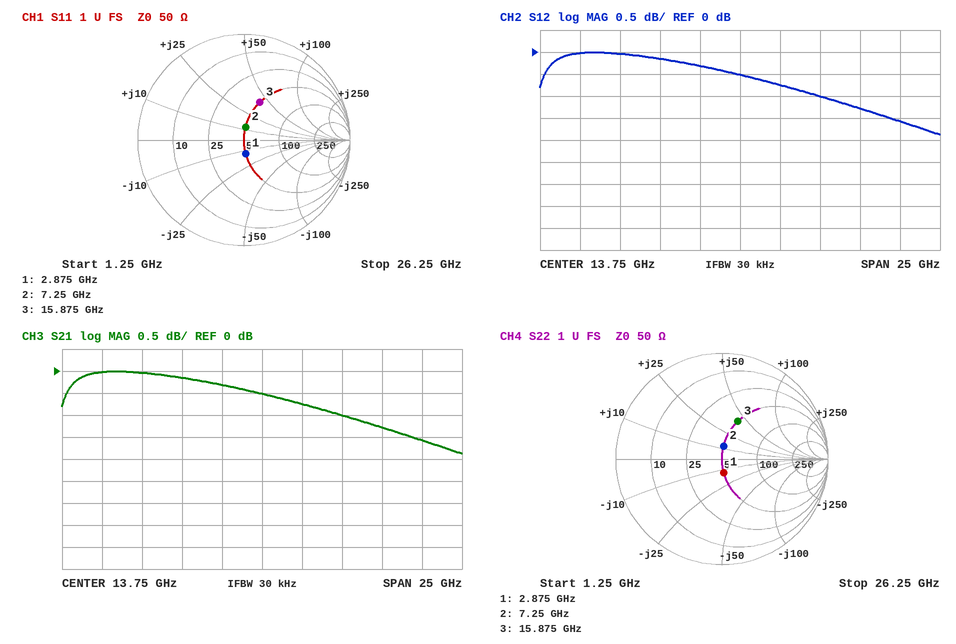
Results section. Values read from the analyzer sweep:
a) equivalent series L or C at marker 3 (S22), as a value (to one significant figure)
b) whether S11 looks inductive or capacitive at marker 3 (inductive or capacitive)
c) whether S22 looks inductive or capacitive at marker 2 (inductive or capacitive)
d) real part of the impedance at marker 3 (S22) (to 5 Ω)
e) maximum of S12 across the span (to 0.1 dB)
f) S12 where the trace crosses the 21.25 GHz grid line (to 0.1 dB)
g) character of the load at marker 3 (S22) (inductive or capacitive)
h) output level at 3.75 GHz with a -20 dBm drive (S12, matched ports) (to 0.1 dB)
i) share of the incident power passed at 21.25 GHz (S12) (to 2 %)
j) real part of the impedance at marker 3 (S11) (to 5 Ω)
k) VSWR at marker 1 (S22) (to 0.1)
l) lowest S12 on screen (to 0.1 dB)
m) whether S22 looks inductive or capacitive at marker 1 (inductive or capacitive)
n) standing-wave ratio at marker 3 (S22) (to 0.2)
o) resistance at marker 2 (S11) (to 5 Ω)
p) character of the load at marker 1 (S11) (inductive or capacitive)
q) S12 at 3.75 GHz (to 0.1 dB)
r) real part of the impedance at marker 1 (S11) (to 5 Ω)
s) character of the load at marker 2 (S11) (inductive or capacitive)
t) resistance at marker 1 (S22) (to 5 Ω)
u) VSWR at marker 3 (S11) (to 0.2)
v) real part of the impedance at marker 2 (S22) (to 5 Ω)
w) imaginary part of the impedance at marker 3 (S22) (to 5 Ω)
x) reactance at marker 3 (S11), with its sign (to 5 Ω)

400 pH
inductive
inductive
50 Ω
0.0 dB
-1.3 dB
inductive
-20.0 dBm
74 %
50 Ω
1.3
-1.9 dB
capacitive
2.2
50 Ω
capacitive
0.0 dB
50 Ω
inductive
50 Ω
2.2
50 Ω
+40 Ω
+40 Ω
